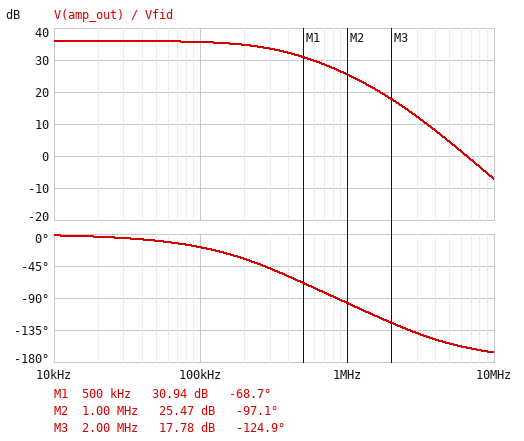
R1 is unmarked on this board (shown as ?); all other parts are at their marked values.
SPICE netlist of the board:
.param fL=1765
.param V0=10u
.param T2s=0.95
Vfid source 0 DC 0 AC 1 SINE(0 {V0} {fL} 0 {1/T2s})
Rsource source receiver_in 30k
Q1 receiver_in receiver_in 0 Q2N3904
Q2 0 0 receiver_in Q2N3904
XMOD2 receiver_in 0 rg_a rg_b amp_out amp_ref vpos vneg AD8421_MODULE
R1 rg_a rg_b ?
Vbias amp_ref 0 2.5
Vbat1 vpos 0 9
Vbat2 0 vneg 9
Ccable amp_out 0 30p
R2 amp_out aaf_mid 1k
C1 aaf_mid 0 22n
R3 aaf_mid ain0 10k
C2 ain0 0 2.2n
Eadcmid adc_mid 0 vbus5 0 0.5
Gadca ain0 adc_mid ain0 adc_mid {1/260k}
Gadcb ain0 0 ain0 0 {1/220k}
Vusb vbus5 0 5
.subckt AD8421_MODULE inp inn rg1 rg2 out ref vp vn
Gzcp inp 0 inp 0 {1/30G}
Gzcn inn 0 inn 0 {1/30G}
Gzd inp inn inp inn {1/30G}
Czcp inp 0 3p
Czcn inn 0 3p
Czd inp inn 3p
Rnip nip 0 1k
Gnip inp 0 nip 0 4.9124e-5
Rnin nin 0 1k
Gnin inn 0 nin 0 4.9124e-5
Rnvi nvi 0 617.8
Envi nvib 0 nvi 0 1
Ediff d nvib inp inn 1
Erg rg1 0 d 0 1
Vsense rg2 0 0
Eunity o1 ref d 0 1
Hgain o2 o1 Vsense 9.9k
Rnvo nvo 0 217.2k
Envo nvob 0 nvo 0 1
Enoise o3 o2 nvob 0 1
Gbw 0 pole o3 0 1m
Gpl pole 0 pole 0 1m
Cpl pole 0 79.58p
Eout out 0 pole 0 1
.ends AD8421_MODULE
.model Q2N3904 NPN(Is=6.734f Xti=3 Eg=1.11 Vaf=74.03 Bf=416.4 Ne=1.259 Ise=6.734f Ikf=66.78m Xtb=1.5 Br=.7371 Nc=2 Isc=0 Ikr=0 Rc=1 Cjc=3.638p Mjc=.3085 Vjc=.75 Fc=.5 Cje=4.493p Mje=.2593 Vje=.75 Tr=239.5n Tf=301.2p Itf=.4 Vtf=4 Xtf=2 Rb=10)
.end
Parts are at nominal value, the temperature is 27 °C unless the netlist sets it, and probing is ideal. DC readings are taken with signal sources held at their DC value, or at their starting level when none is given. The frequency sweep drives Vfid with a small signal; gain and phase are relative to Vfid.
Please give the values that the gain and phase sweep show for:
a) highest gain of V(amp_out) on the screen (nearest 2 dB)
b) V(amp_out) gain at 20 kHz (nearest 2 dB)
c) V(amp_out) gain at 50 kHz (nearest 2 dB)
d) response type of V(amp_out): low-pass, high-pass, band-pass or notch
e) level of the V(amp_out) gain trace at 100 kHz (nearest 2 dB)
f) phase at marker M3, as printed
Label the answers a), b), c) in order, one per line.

a) 36 dB
b) 36 dB
c) 36 dB
d) low-pass
e) 36 dB
f) -124.9 deg
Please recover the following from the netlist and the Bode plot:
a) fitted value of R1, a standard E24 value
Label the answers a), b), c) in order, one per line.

a) 160 Ω
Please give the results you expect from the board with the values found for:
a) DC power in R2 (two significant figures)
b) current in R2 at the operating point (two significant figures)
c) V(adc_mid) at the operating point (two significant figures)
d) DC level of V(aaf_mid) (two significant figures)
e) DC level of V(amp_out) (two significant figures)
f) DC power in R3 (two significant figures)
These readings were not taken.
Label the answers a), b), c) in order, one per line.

a) 110 nW
b) 10 µA
c) 2.5 V
d) 2.5 V
e) 2.5 V
f) 1.1 µW
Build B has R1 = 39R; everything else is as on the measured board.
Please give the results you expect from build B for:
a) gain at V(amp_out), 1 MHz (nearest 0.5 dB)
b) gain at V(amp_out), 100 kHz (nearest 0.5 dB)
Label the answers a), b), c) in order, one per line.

a) 37.5 dB
b) 48.0 dB
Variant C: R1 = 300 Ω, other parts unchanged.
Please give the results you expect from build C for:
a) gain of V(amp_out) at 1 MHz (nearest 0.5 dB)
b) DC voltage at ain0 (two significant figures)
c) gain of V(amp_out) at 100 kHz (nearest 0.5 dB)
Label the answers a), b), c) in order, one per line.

a) 20.0 dB
b) 2.4 V
c) 30.5 dB
